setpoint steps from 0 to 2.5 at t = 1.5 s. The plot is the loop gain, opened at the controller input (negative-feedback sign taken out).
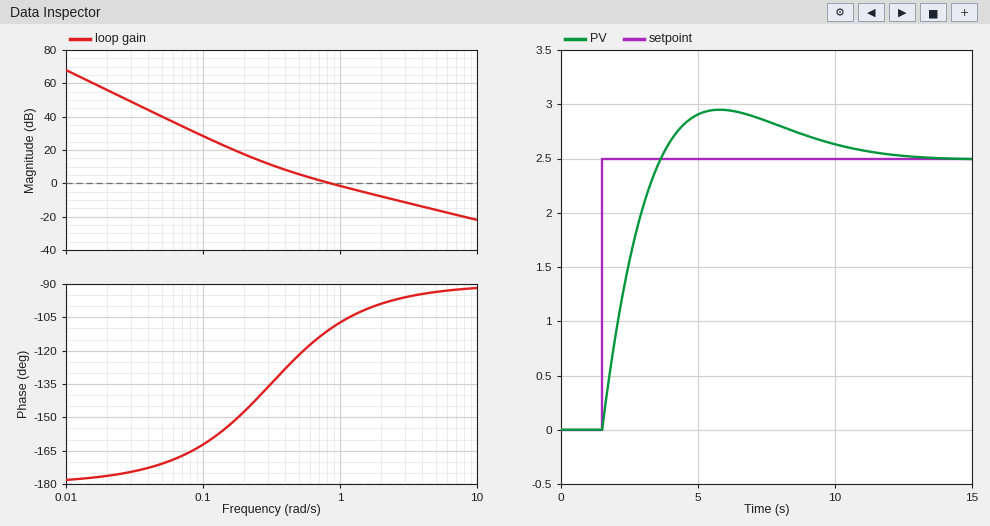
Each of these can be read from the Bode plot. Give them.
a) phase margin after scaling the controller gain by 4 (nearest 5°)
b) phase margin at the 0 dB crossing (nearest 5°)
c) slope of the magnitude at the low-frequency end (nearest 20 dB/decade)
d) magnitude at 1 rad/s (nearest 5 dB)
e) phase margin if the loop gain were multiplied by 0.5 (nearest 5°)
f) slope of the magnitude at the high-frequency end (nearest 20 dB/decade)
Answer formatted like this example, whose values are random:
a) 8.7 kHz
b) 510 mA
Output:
a) 85°
b) 70°
c) -40 dB/decade
d) 0 dB
e) 55°
f) -20 dB/decade
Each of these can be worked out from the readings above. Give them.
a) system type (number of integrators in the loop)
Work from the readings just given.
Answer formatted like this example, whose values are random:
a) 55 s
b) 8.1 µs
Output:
a) 2
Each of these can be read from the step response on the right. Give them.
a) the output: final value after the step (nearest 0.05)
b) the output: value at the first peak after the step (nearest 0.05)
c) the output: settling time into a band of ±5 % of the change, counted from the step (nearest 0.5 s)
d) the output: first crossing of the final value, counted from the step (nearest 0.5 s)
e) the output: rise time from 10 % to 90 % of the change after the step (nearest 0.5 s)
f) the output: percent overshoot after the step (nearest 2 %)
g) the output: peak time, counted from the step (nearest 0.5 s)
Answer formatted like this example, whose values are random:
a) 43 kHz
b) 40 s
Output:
a) 2.50
b) 2.95
c) 8.5 s
d) 2.0 s
e) 1.5 s
f) 18 %
g) 4.5 s
